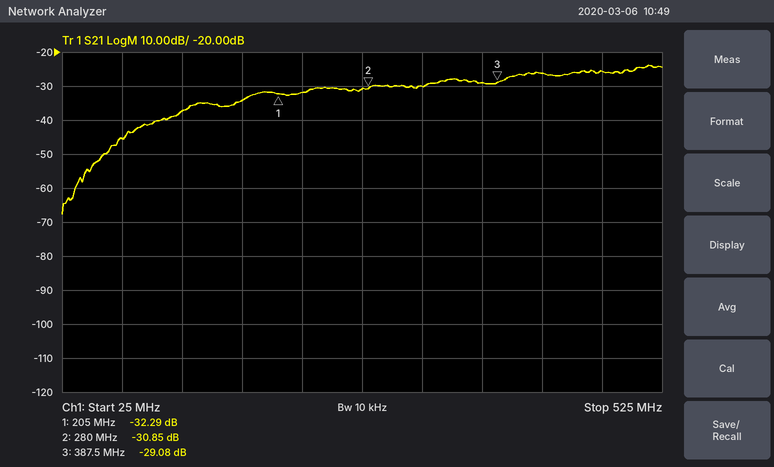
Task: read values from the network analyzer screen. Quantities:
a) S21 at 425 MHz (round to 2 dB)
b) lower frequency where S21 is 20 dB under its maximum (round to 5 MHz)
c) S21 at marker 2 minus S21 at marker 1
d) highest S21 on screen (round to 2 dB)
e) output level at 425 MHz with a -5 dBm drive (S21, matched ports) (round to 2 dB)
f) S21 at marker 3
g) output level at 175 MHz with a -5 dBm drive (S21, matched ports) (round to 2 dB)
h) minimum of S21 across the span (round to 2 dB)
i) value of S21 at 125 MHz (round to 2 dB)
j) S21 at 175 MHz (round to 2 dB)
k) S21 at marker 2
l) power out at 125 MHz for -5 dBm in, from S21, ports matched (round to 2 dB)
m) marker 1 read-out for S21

-26 dB
80 MHz
1.44 dB
-24 dB
-32 dBm
-29.08 dB
-40 dBm
-68 dB
-38 dB
-34 dB
-30.85 dB
-42 dBm
-32.29 dB
